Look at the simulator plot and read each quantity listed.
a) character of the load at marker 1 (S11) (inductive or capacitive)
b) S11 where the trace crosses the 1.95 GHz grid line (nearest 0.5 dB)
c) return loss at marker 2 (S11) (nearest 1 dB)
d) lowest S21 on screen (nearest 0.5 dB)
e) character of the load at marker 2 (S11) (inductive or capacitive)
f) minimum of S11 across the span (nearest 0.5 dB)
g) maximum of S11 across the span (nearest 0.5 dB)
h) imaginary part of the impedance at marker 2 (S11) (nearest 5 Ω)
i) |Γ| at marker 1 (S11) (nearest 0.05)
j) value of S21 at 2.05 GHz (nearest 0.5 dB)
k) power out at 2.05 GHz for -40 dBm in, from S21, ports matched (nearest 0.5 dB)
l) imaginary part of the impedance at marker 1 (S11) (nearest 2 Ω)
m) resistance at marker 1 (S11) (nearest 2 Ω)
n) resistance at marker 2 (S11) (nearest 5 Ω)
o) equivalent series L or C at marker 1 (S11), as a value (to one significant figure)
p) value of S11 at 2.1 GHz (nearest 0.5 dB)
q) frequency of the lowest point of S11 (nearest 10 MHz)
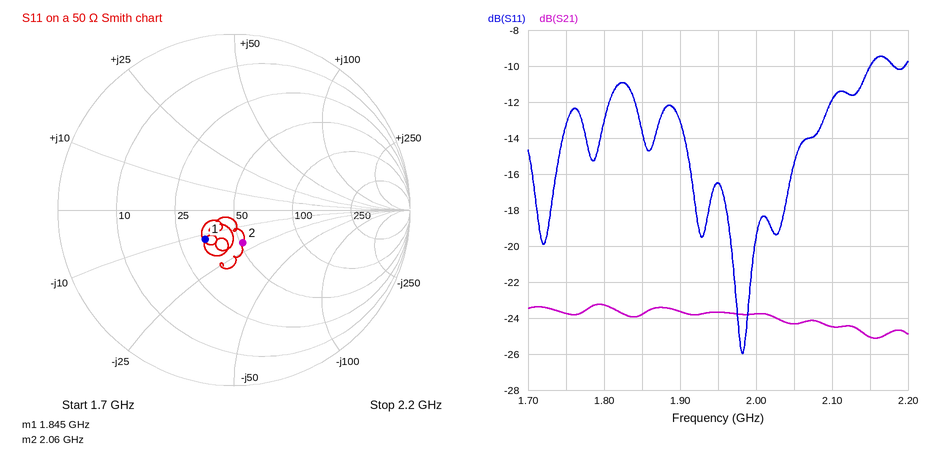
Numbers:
capacitive
-16.5 dB
14 dB
-25.0 dB
capacitive
-26.0 dB
-9.5 dB
-20 Ω
0.25
-24.5 dB
-64.5 dBm
-12 Ω
34 Ω
50 Ω
7 pF
-12.0 dB
1.98 GHz
